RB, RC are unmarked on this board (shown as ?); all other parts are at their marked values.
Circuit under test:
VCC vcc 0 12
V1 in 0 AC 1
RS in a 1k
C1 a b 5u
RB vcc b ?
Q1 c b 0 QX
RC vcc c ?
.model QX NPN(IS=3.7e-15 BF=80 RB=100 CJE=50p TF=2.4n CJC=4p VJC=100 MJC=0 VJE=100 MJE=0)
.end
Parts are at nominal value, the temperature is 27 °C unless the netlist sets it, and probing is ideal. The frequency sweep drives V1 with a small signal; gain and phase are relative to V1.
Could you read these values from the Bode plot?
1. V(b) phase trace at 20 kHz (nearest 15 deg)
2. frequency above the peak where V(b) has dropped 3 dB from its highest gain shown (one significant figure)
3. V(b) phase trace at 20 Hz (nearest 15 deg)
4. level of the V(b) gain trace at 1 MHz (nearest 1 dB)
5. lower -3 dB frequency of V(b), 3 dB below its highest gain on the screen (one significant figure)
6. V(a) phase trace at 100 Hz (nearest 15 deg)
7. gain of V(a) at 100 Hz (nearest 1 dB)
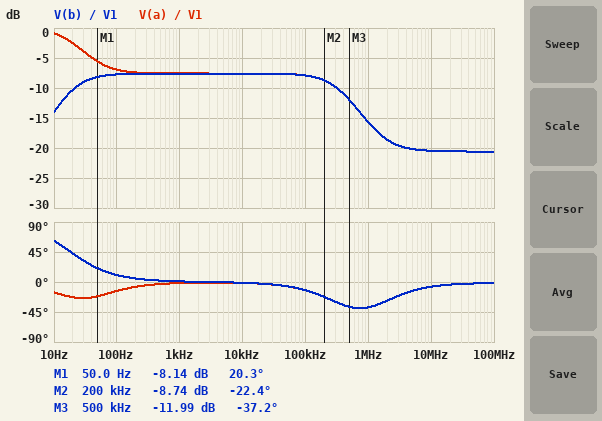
0 deg
400 kHz
45 deg
-16 dB
20 Hz
-15 deg
-7 dB
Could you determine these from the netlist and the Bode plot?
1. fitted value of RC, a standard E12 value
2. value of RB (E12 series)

1.5 kΩ
270 kΩ
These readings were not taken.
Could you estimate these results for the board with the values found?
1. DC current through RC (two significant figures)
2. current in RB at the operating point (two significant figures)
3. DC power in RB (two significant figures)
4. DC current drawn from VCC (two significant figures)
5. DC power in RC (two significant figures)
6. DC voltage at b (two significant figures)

3.3 mA
42 µA
470 µW
3.4 mA
17 mW
720 mV
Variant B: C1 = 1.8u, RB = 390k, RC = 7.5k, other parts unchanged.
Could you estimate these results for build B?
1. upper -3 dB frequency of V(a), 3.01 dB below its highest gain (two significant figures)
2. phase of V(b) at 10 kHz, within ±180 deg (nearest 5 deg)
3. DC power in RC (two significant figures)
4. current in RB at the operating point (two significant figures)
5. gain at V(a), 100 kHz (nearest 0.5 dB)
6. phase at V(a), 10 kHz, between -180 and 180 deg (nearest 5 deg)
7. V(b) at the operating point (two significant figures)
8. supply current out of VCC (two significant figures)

79 Hz
0 deg
19 mW
29 µA
-18.5 dB
-5 deg
700 mV
1.6 mA
